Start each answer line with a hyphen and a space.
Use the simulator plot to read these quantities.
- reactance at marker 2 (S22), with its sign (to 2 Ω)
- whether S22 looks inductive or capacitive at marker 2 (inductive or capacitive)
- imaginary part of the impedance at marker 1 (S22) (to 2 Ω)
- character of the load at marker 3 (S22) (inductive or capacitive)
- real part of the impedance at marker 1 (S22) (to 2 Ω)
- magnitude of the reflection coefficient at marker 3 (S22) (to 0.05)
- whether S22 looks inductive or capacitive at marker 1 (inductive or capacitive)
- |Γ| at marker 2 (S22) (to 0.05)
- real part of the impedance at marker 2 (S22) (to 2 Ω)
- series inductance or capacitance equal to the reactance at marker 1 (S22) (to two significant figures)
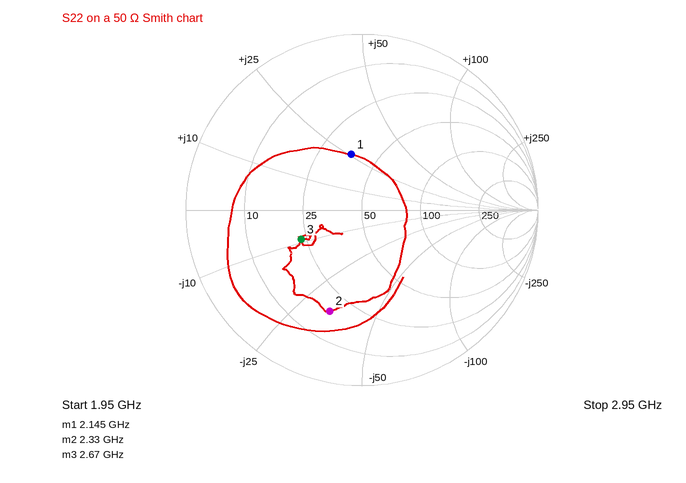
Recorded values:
- -34 Ω
- capacitive
- +26 Ω
- capacitive
- 36 Ω
- 0.40
- inductive
- 0.60
- 18 Ω
- 1.9 nH
